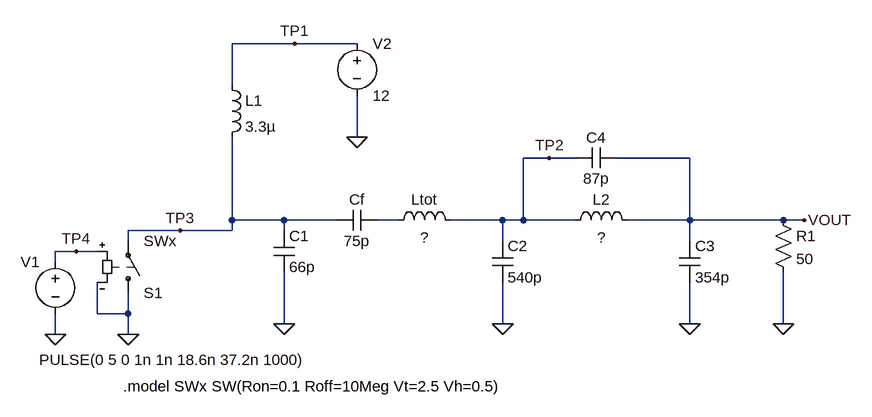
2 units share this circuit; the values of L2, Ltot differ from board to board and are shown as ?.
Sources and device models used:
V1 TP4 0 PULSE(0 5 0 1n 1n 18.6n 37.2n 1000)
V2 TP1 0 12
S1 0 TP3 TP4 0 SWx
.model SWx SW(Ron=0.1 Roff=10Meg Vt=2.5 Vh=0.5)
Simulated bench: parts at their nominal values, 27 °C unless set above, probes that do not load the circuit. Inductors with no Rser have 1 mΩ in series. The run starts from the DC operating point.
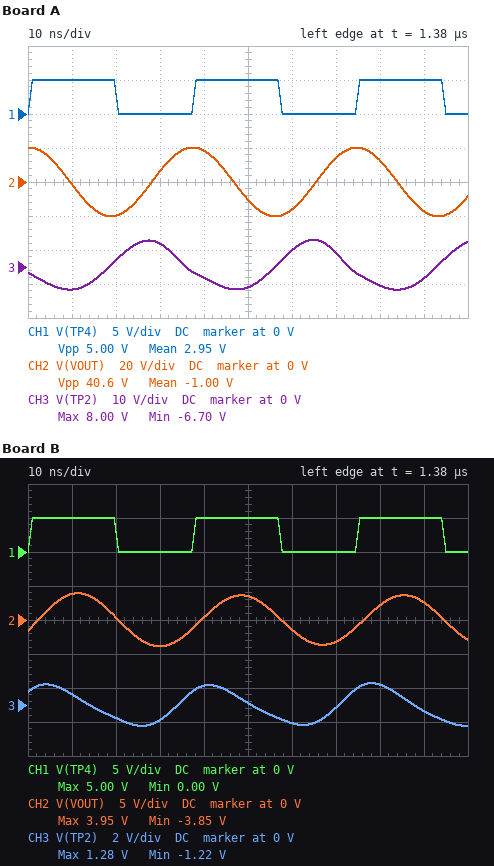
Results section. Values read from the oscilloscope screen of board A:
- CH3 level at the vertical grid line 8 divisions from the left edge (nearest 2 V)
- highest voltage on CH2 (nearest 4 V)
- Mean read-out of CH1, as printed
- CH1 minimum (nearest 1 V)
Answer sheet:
-6 V
20 V
2.95 V
0 V
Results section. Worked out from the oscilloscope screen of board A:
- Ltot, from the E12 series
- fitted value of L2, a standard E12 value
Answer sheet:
390 nH
82 nH
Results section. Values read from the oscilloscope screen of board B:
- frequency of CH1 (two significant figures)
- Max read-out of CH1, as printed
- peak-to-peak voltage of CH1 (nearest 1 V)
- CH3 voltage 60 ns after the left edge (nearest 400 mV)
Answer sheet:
27 MHz
5.00 V
5 V
-1.2 V
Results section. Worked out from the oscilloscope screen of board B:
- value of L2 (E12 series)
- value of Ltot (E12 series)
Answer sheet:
68 nH
820 nH
